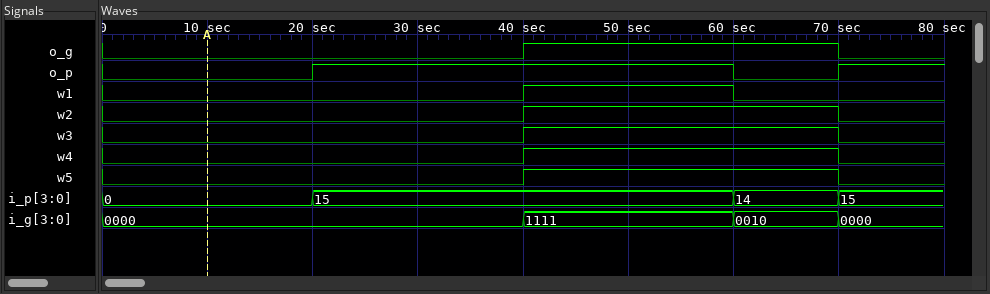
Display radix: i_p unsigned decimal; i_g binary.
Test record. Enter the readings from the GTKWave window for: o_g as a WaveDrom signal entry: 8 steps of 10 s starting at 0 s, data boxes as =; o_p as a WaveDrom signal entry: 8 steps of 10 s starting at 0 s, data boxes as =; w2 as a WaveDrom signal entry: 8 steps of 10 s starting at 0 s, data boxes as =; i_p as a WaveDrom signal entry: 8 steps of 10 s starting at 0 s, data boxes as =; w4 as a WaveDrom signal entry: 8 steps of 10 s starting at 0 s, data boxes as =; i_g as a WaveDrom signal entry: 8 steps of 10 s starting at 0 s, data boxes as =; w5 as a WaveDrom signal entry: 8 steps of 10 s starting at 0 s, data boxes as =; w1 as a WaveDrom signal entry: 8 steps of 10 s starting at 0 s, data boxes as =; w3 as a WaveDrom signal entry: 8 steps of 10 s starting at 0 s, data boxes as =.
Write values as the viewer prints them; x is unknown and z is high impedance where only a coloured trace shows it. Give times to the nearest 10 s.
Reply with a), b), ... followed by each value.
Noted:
a) {name: 'o_g', wave: '0...1..0'}
b) {name: 'o_p', wave: '0.1...01'}
c) {name: 'w2', wave: '0...1..0'}
d) {name: 'i_p', wave: '=.=...==', data: '0 15 14 15'}
e) {name: 'w4', wave: '0...1..0'}
f) {name: 'i_g', wave: '=...=.==', data: '0000 1111 0010 0000'}
g) {name: 'w5', wave: '0...1..0'}
h) {name: 'w1', wave: '0...1.0.'}
i) {name: 'w3', wave: '0...1..0'}
